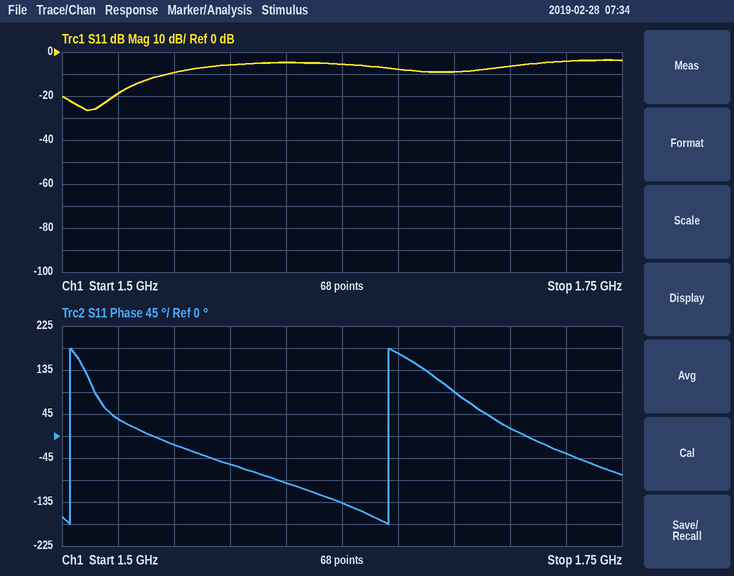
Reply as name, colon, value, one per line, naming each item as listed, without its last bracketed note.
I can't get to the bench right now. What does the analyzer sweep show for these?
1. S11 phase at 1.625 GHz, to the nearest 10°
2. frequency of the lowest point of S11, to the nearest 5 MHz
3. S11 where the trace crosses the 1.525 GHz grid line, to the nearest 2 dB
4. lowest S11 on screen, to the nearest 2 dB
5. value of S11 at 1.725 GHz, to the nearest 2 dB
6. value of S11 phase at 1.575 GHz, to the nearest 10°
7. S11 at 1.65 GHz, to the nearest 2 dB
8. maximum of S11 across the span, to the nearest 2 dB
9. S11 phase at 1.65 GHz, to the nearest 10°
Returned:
S11 phase at 1.625 GHz, to the nearest 10°: -140°
frequency of the lowest point of S11, to the nearest 5 MHz: 1.510 GHz
S11 where the trace crosses the 1.525 GHz grid line, to the nearest 2 dB: -18 dB
lowest S11 on screen, to the nearest 2 dB: -26 dB
value of S11 at 1.725 GHz, to the nearest 2 dB: -4 dB
value of S11 phase at 1.575 GHz, to the nearest 10°: -60°
S11 at 1.65 GHz, to the nearest 2 dB: -8 dB
maximum of S11 across the span, to the nearest 2 dB: -4 dB
S11 phase at 1.65 GHz, to the nearest 10°: 170°
